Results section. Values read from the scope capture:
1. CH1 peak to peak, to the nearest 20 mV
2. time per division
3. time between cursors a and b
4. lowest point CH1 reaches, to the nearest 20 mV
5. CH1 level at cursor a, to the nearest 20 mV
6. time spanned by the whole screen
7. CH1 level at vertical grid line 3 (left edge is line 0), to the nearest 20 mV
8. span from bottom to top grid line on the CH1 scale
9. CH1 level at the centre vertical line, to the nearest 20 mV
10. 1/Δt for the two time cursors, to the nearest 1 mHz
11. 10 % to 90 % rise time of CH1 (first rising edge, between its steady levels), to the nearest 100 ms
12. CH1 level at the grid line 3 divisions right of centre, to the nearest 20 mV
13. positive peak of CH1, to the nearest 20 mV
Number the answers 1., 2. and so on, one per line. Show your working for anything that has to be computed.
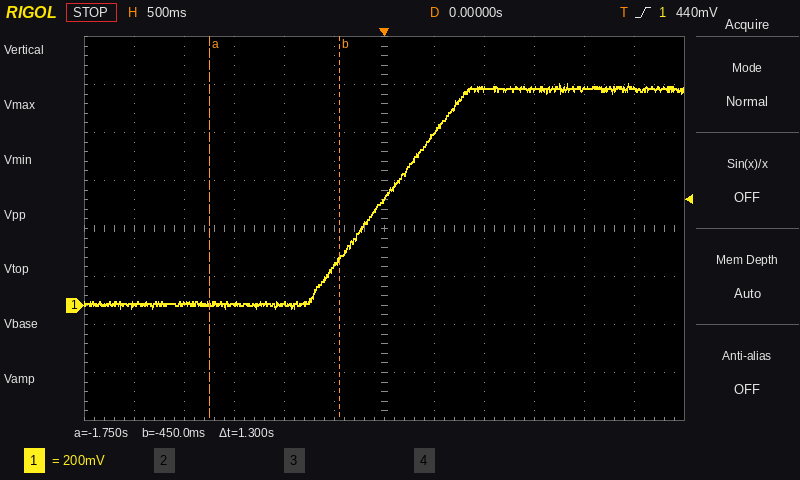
1. 920 mV − (-20 mV) = 940 mV
2. 500 ms
3. 1.3 s
4. -20 mV
5. 0 mV
6. 6 s
7. 0 mV
8. 1.6 V
9. 440 mV
10. 1 / 1.3 s ≈ 769 mHz
11. 1.3 s
12. 900 mV
13. 920 mV
